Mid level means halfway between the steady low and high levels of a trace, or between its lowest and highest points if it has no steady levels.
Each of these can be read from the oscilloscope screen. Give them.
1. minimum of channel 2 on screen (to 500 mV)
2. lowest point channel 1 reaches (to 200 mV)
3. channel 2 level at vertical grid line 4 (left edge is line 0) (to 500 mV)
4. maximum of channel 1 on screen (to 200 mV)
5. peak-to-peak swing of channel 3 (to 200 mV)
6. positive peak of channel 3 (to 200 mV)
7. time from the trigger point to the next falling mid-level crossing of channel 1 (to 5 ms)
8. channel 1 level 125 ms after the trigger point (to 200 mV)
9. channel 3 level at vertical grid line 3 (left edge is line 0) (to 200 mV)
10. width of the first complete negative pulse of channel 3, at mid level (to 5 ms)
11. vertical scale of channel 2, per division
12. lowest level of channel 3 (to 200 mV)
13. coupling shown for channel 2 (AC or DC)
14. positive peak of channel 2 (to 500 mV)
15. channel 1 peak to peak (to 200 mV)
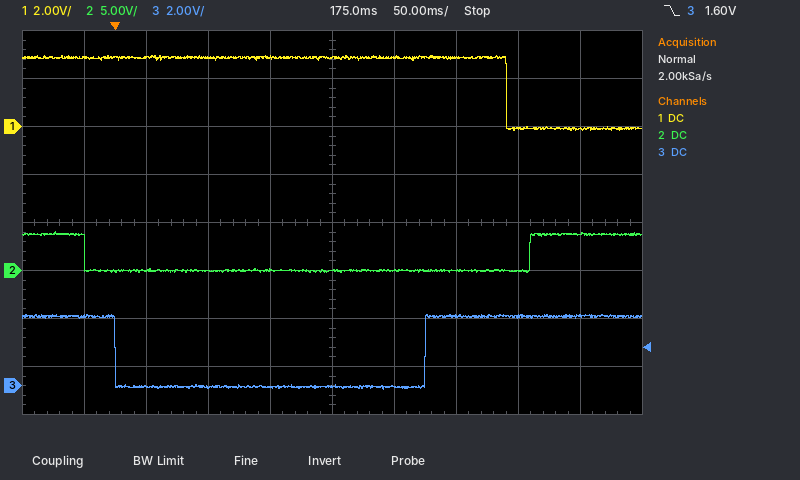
0.0 V
-200 mV
0.0 V
3.0 V
3.2 V
3.0 V
315 ms
2.8 V
0.0 V
250 ms
5 V
-200 mV
DC
4.0 V
3.2 V
